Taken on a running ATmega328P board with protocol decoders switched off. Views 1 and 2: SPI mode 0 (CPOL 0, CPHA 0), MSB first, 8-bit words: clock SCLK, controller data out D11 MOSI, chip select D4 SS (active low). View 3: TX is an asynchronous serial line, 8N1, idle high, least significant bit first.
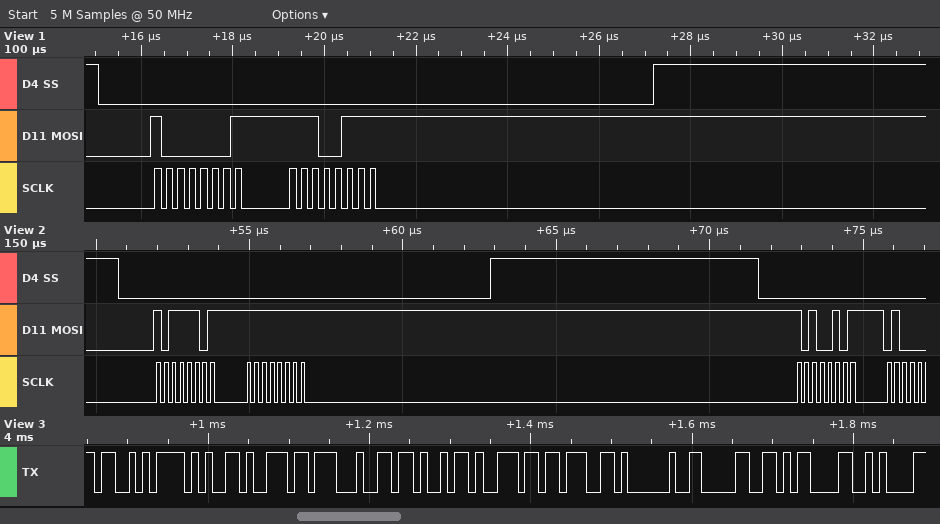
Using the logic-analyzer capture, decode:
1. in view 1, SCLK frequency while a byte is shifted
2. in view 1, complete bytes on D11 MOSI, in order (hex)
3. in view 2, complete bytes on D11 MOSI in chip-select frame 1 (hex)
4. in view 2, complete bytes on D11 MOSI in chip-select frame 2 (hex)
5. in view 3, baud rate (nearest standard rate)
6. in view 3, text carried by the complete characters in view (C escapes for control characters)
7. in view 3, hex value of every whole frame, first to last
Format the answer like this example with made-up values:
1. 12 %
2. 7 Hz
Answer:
1. 4 MHz
2. 0x81 0xE7
3. BD FF
4. A5
5. 115200 baud
6. "Sending 0\r\n"
7. 53 65 6E 64 69 6E 67 20 30 0D 0A
